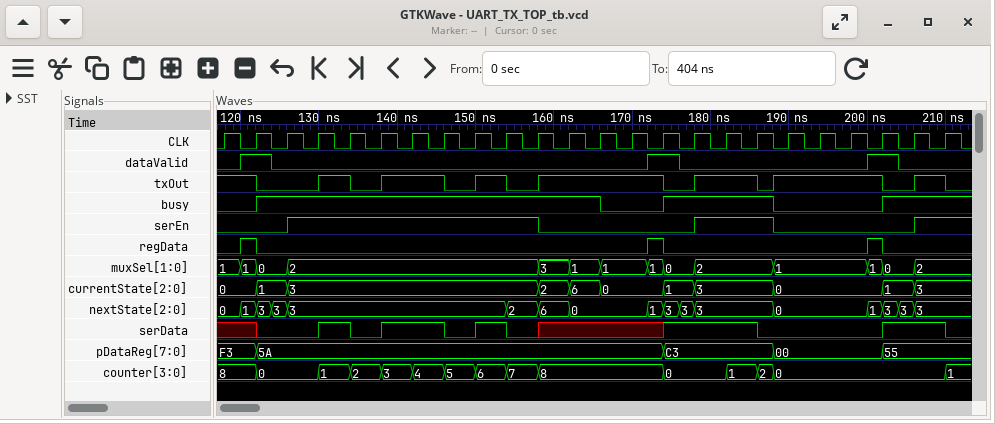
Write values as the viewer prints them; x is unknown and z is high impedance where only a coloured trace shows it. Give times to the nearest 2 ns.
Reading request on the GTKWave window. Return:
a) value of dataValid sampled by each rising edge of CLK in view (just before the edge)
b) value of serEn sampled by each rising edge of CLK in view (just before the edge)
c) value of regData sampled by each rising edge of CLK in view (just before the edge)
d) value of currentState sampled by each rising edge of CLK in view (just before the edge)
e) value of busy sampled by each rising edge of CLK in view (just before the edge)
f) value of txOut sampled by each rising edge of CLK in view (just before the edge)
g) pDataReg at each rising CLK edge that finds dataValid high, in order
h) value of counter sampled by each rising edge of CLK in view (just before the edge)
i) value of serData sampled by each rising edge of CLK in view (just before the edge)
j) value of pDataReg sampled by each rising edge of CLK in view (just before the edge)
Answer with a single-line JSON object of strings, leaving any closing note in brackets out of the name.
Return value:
{"value of dataValid sampled by each rising edge of CLK in view": "0 1 0 0 0 0 0 0 0 0 0 0 0 0 1 0 0 0 0 0 0 1 0 0", "value of serEn sampled by each rising edge of CLK in view": "0 0 0 1 1 1 1 1 1 1 1 0 0 0 0 0 1 1 0 0 0 0 0 1", "value of regData sampled by each rising edge of CLK in view": "0 1 0 0 0 0 0 0 0 0 0 0 0 0 1 0 0 0 0 0 0 1 0 0", "value of currentState sampled by each rising edge of CLK in view": "0, 0, 1, 3, 3, 3, 3, 3, 3, 3, 3, 2, 6, 0, 0, 1, 3, 3, 0, 0, 0, 0, 1, 3", "value of busy sampled by each rising edge of CLK in view": "0 0 1 1 1 1 1 1 1 1 1 1 1 0 0 1 1 1 0 0 0 0 1 1", "value of txOut sampled by each rising edge of CLK in view": "1 1 0 0 1 0 1 1 0 1 0 1 1 1 1 0 1 1 1 1 1 1 0 1", "pDataReg at each rising CLK edge that finds dataValid high, in order": "F3, 5A, 00", "value of counter sampled by each rising edge of CLK in view": "8, 8, 0, 0, 1, 2, 3, 4, 5, 6, 7, 8, 8, 8, 8, 0, 0, 1, 0, 0, 0, 0, 0, 0", "value of serData sampled by each rising edge of CLK in view": "x x 0 0 1 0 1 1 0 1 0 x x x x 1 1 1 0 0 0 0 1 1", "value of pDataReg sampled by each rising edge of CLK in view": "F3, F3, 5A, 5A, 5A, 5A, 5A, 5A, 5A, 5A, 5A, 5A, 5A, 5A, 5A, C3, C3, C3, 00, 00, 00, 00, 55, 55"}
